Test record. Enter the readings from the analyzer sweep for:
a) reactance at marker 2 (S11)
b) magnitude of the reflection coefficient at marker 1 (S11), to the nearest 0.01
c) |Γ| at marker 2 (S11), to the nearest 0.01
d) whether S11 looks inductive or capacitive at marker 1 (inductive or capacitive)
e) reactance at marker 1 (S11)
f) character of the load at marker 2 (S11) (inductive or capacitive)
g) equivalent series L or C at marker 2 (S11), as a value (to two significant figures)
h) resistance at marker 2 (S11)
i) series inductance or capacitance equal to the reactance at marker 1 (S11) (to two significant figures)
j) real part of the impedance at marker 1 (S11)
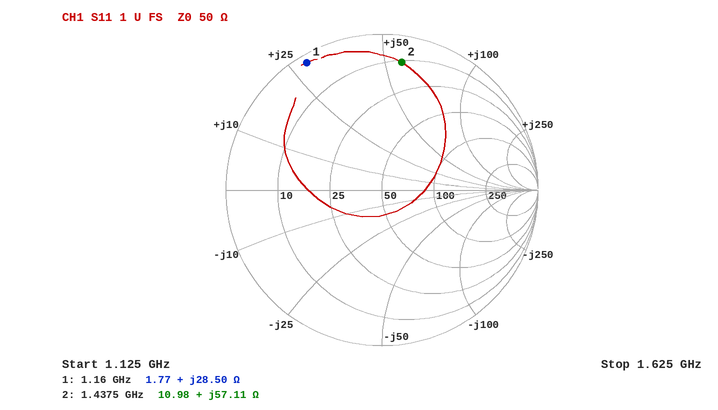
+57.11 Ω
0.95
0.83
inductive
+28.50 Ω
inductive
6.3 nH
10.98 Ω
3.9 nH
1.77 Ω
